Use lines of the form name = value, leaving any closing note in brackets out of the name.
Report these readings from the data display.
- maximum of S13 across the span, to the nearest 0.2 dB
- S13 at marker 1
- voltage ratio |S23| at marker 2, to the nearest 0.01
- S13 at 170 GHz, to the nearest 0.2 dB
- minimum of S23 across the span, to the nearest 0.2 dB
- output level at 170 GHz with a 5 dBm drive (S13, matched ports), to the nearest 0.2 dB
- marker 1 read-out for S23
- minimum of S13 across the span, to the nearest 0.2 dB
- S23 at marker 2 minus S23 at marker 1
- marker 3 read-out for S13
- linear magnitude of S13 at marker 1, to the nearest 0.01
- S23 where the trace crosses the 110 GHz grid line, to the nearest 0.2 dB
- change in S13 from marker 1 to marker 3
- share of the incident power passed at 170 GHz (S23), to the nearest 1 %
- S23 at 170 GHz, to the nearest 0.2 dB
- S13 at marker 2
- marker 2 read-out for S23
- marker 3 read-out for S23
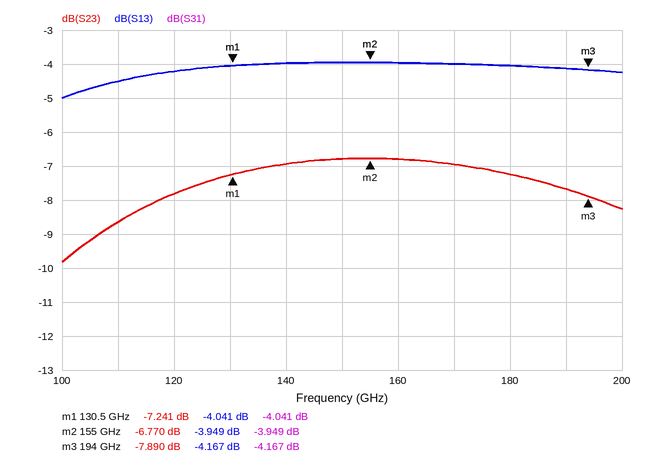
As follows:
maximum of S13 across the span, to the nearest 0.2 dB = -4.0 dB
S13 at marker 1 = -4.041 dB
voltage ratio |S23| at marker 2, to the nearest 0.01 = 0.46
S13 at 170 GHz, to the nearest 0.2 dB = -4.0 dB
minimum of S23 across the span, to the nearest 0.2 dB = -9.8 dB
output level at 170 GHz with a 5 dBm drive (S13, matched ports), to the nearest 0.2 dB = 1.0 dBm
marker 1 read-out for S23 = -7.241 dB
minimum of S13 across the span, to the nearest 0.2 dB = -5.0 dB
S23 at marker 2 minus S23 at marker 1 = 0.471 dB
marker 3 read-out for S13 = -4.167 dB
linear magnitude of S13 at marker 1, to the nearest 0.01 = 0.63
S23 where the trace crosses the 110 GHz grid line, to the nearest 0.2 dB = -8.6 dB
change in S13 from marker 1 to marker 3 = -0.126 dB
share of the incident power passed at 170 GHz (S23), to the nearest 1 % = 20 %
S23 at 170 GHz, to the nearest 0.2 dB = -7.0 dB
S13 at marker 2 = -3.949 dB
marker 2 read-out for S23 = -6.770 dB
marker 3 read-out for S23 = -7.890 dB
